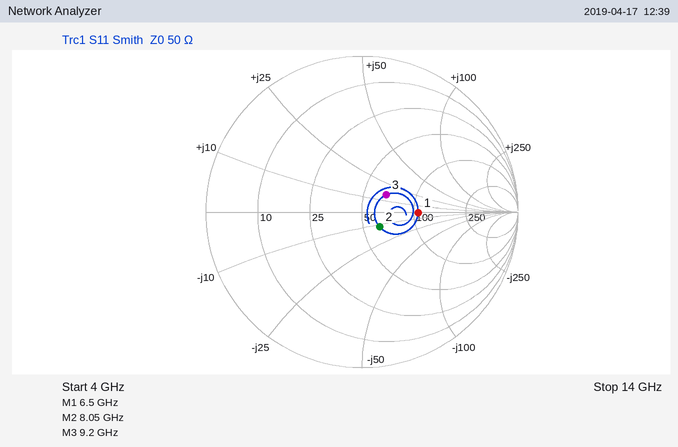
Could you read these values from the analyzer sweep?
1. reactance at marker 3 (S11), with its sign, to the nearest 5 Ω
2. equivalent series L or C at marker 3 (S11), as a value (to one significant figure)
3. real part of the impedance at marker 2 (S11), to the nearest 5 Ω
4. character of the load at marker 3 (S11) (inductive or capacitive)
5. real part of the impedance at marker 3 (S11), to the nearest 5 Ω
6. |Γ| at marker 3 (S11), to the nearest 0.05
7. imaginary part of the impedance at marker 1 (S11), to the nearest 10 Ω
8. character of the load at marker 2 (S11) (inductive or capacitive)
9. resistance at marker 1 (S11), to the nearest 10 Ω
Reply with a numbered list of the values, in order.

1. +15 Ω
2. 300 pH
3. 60 Ω
4. inductive
5. 65 Ω
6. 0.20
7. 0 Ω
8. capacitive
9. 110 Ω
